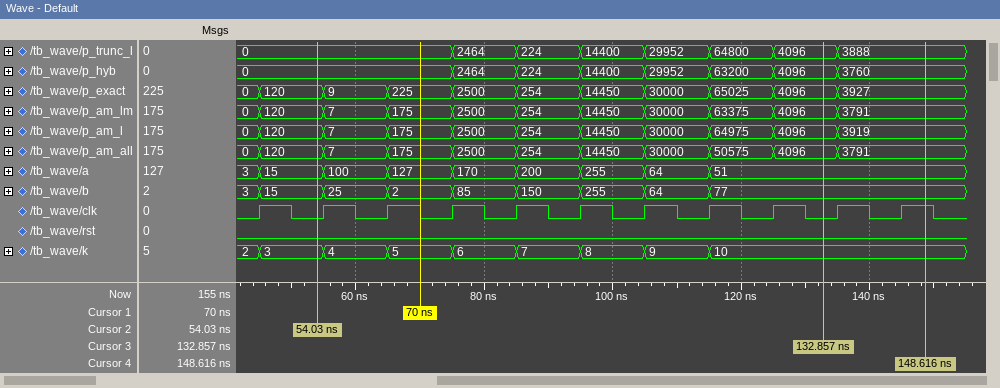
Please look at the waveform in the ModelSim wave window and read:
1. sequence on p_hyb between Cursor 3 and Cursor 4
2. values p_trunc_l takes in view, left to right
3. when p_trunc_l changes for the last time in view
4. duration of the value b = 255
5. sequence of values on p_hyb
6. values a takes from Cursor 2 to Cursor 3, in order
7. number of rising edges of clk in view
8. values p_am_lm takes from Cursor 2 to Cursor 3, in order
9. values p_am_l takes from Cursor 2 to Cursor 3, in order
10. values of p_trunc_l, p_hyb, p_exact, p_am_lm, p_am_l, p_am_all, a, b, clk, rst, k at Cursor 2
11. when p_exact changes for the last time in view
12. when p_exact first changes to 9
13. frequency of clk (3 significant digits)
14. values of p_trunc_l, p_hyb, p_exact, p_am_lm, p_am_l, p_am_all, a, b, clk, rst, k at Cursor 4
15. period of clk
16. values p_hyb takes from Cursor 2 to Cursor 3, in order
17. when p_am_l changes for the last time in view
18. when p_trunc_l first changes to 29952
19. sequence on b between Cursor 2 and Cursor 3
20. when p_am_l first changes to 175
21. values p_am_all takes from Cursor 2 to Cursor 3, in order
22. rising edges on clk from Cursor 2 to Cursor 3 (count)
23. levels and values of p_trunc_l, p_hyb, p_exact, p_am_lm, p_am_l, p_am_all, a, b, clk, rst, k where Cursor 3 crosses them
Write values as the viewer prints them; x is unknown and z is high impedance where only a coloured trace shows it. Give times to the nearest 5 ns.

4096, 3760
0, 2464, 224, 14400, 29952, 64800, 4096, 3888
135 ns
10 ns
0, 2464, 224, 14400, 29952, 63200, 4096, 3760
15, 100, 127, 170, 200, 255, 64, 51
11
120, 7, 175, 2500, 254, 14450, 30000, 63375, 4096
120, 7, 175, 2500, 254, 14450, 30000, 64975, 4096
p_trunc_l=0, p_hyb=0, p_exact=120, p_am_lm=120, p_am_l=120, p_am_all=120, a=15, b=15, clk=0, rst=0, k=3
135 ns
55 ns
100 MHz
p_trunc_l=3888, p_hyb=3760, p_exact=3927, p_am_lm=3791, p_am_l=3919, p_am_all=3791, a=51, b=77, clk=1, rst=0, k=10
10 ns
0, 2464, 224, 14400, 29952, 63200, 4096
135 ns
105 ns
15, 25, 2, 85, 150, 255, 64, 77
65 ns
120, 7, 175, 2500, 254, 14450, 30000, 50575, 4096
8
p_trunc_l=4096, p_hyb=4096, p_exact=4096, p_am_lm=4096, p_am_l=4096, p_am_all=4096, a=51, b=77, clk=0, rst=0, k=10
